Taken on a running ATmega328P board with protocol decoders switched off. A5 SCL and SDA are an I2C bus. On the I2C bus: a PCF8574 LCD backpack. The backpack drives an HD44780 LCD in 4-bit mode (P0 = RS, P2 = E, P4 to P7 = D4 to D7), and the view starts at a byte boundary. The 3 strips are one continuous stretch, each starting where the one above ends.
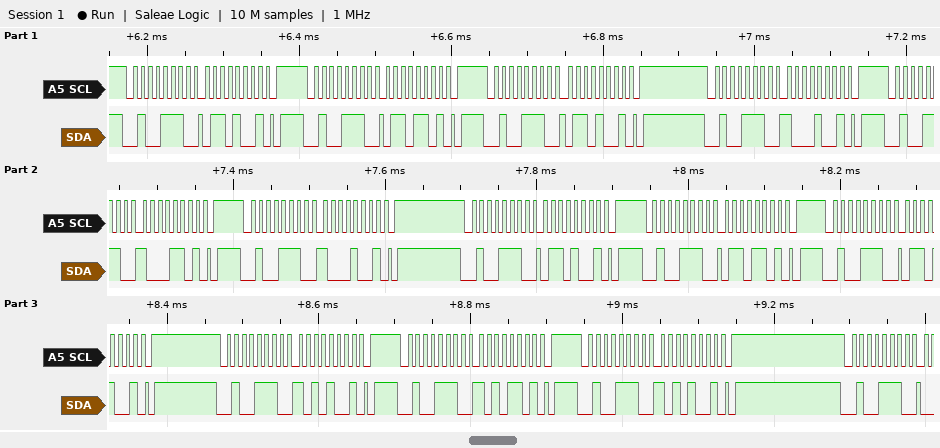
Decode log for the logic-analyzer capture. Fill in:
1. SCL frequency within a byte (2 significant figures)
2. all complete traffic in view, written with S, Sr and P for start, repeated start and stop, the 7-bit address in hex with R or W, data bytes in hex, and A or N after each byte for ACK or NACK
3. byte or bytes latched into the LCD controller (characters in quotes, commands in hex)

100 kHz
S 27W A 69 A P S 27W A 6D A P S 27W A 69 A P S 27W A 89 A P S 27W A 8D A P S 27W A 89 A P S 27W A 69 A P S 27W A 6D A P S 27W A 69 A P S 27W A A9 A P S 27W A AD A P S 27W A A9 A P S 27W A
'h' 'j'
